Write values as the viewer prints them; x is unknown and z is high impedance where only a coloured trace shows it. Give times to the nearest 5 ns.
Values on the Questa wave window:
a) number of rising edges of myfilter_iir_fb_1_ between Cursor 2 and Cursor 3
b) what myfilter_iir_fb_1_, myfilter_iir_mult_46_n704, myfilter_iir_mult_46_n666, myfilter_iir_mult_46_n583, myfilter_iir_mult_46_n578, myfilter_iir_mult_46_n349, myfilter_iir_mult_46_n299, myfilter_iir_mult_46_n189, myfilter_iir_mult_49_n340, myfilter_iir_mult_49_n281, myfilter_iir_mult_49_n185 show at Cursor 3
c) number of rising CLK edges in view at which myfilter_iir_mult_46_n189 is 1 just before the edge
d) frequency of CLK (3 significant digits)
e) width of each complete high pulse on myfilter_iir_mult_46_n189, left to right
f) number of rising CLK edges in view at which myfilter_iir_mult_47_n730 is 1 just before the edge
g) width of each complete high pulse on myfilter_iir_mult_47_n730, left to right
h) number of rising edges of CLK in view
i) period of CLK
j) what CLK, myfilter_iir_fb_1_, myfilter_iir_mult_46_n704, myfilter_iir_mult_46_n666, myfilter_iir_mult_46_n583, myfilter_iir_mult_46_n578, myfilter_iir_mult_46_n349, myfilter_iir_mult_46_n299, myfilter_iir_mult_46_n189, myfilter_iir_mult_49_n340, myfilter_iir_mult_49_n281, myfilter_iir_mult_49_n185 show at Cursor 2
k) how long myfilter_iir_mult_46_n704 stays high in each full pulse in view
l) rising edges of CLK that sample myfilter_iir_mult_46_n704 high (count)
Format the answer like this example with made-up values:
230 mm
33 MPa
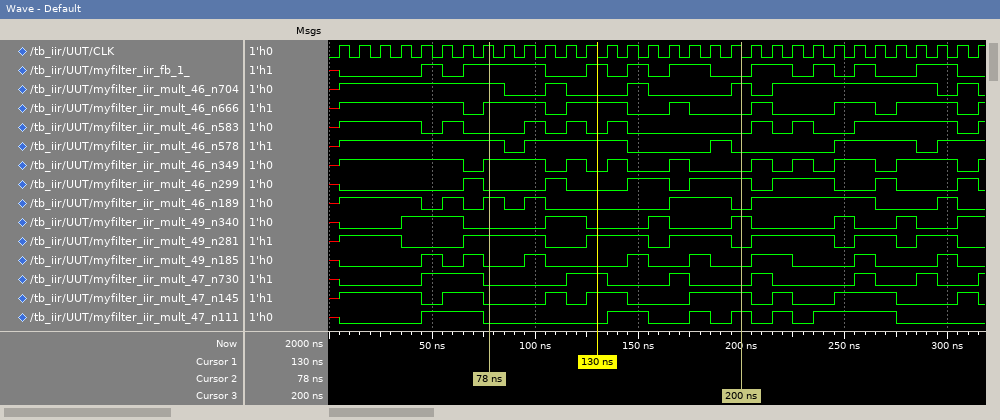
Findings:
3
myfilter_iir_fb_1_=0, myfilter_iir_mult_46_n704=1, myfilter_iir_mult_46_n666=0, myfilter_iir_mult_46_n583=0, myfilter_iir_mult_46_n578=0, myfilter_iir_mult_46_n349=0, myfilter_iir_mult_46_n299=1, myfilter_iir_mult_46_n189=0, myfilter_iir_mult_49_n340=1, myfilter_iir_mult_49_n281=0, myfilter_iir_mult_49_n185=0
17
100 MHz
10 ns, 10 ns, 10 ns, 30 ns, 60 ns, 10 ns
9
30 ns, 20 ns, 10 ns, 10 ns, 10 ns, 10 ns
32
10 ns
CLK=1, myfilter_iir_fb_1_=1, myfilter_iir_mult_46_n704=1, myfilter_iir_mult_46_n666=1, myfilter_iir_mult_46_n583=0, myfilter_iir_mult_46_n578=1, myfilter_iir_mult_46_n349=1, myfilter_iir_mult_46_n299=0, myfilter_iir_mult_46_n189=1, myfilter_iir_mult_49_n340=0, myfilter_iir_mult_49_n281=1, myfilter_iir_mult_49_n185=0
10 ns, 10 ns, 10 ns, 80 ns, 10 ns
20
